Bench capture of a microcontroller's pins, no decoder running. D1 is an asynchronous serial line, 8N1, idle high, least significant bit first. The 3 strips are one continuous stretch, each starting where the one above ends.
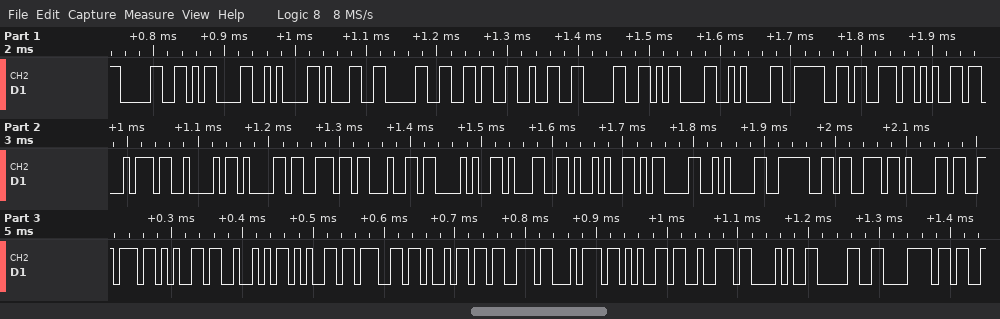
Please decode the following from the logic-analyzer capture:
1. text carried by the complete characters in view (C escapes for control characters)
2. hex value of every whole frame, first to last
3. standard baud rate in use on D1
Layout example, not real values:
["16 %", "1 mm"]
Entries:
["\"0\\r\\n10620\\r\\n>setBand(1)\\r\\n>saveRegister(0x\"", "30 0D 0A 31 30 36 32 30 0D 0A 3E 73 65 74 42 61 6E 64 28 31 29 0D 0A 3E 73 61 76 65 52 65 67 69 73 74 65 72 28 30 78", "115200 baud"]
